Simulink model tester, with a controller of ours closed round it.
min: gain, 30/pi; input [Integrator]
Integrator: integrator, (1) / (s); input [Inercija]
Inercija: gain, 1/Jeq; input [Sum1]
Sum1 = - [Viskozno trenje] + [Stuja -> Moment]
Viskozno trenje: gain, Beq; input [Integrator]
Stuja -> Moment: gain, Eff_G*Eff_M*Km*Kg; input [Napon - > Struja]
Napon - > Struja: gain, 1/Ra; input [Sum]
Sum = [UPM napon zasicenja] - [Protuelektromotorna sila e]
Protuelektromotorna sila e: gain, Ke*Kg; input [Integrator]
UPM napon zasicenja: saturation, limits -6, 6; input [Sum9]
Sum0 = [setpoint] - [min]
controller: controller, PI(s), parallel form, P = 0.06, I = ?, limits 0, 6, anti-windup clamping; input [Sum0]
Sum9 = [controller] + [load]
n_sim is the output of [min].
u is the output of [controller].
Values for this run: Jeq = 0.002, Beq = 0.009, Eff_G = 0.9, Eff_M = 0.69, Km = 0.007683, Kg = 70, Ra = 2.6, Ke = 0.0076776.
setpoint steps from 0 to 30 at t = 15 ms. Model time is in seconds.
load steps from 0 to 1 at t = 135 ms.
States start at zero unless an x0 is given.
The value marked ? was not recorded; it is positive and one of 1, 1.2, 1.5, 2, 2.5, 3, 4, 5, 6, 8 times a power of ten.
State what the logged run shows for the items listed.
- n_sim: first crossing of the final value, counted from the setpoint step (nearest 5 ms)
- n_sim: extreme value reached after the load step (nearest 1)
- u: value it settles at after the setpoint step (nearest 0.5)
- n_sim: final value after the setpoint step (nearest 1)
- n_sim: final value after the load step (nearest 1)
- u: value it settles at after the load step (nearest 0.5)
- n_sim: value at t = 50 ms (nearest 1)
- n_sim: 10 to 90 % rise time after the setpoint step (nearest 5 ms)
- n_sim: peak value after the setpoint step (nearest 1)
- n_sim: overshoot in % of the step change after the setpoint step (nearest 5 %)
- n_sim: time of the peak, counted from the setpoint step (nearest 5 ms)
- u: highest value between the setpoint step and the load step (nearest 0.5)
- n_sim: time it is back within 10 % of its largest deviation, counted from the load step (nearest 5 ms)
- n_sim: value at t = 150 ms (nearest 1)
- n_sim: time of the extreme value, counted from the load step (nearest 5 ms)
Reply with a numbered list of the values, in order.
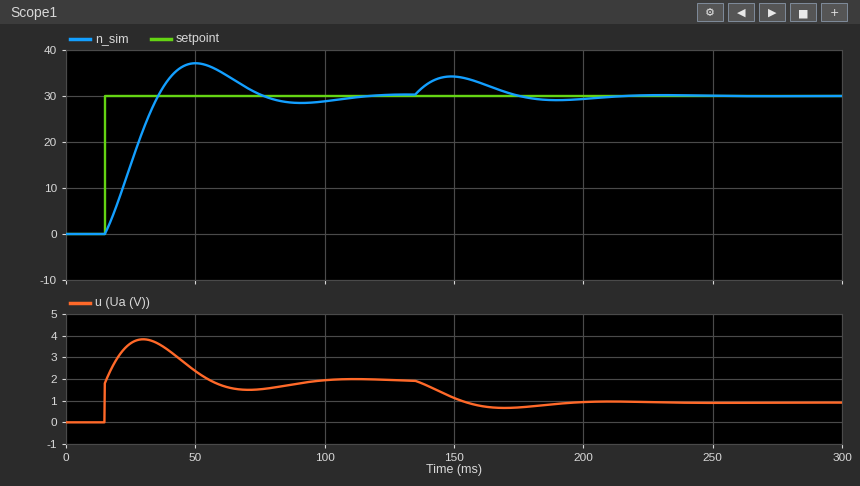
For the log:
1. 20 ms
2. 34
3. 2.0
4. 30
5. 30
6. 1.0
7. 37
8. 15 ms
9. 37
10. 25 %
11. 35 ms
12. 4.0
13. 70 ms
14. 34
15. 15 ms
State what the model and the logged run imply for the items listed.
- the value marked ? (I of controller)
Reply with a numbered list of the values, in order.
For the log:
1. 12
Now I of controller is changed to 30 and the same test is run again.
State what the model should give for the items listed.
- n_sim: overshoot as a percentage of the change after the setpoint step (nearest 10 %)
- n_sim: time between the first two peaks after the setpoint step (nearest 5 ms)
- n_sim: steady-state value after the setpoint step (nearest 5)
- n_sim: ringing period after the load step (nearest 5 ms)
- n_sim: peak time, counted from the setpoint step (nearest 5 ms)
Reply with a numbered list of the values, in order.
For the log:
1. 40 %
2. 50 ms
3. 30
4. 50 ms
5. 20 ms
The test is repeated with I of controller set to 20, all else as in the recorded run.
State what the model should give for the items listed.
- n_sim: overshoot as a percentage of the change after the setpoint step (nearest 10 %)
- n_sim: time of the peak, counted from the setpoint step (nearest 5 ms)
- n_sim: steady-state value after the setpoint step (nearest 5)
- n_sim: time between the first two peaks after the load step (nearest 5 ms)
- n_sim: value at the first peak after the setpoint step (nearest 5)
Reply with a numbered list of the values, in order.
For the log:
1. 30 %
2. 25 ms
3. 30
4. 60 ms
5. 40
